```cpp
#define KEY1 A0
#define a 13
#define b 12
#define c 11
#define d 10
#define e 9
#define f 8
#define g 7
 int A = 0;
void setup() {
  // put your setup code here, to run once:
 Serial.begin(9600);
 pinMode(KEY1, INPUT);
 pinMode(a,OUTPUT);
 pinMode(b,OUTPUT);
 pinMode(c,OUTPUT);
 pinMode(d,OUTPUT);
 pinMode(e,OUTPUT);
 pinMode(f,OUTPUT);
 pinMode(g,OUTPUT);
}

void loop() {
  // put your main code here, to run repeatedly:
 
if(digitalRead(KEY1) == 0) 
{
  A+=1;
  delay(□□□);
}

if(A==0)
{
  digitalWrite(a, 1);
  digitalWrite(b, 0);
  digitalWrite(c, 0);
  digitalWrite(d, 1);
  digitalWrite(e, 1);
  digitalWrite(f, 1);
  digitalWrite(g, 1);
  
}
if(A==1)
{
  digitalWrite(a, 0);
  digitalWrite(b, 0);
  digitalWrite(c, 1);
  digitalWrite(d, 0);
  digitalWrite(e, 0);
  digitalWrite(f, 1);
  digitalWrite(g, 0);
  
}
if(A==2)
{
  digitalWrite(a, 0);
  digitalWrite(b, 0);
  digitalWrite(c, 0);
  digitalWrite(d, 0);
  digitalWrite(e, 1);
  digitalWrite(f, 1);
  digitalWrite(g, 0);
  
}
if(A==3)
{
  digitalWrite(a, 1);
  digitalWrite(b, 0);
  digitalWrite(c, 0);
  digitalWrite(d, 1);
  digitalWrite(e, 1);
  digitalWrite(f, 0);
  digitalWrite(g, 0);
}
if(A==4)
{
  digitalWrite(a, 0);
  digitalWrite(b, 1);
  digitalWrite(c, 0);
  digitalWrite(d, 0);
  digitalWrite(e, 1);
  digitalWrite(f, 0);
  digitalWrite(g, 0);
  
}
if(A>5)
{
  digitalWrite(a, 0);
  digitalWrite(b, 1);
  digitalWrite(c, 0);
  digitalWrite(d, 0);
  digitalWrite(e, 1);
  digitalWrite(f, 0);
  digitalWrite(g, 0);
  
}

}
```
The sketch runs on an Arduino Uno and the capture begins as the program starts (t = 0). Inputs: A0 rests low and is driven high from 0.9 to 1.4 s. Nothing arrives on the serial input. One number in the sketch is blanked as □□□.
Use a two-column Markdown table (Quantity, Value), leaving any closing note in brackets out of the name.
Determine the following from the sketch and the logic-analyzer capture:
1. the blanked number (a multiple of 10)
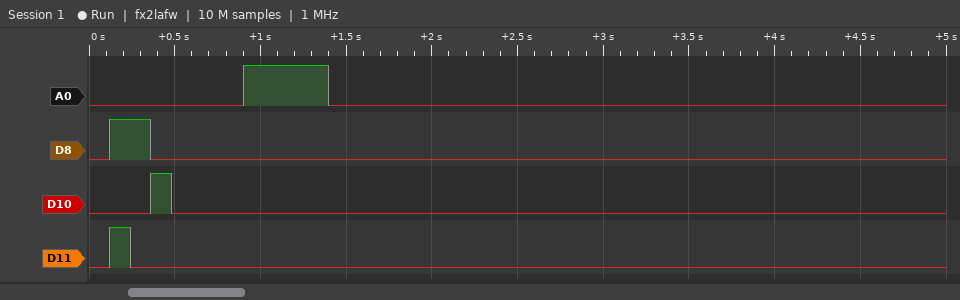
| Quantity | Value |
|---|---|
| the blanked number | 120 |
